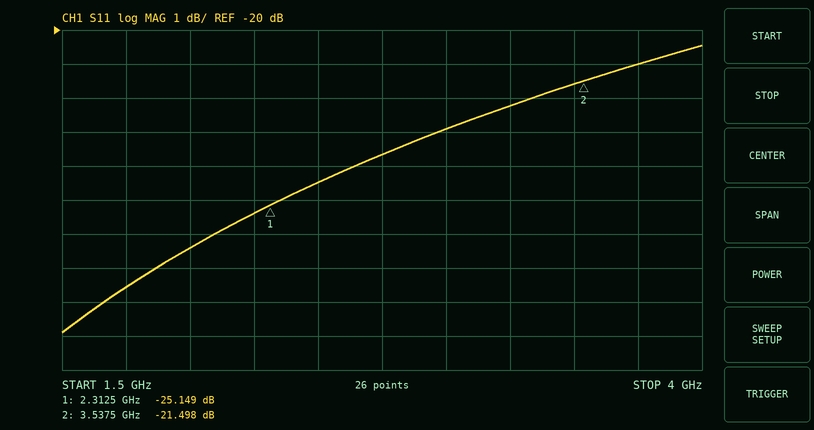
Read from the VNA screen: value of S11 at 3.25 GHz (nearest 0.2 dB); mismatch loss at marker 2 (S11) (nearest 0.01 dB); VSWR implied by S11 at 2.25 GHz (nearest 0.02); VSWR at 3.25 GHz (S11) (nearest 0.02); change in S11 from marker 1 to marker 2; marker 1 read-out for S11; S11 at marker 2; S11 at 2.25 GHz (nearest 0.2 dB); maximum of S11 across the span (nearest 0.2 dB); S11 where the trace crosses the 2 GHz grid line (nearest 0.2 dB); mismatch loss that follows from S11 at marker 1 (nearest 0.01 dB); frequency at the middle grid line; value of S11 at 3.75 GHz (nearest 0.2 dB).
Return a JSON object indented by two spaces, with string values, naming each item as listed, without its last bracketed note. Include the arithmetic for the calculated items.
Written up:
{
  "value of S11 at 3.25 GHz": "-22.2 dB",
  "mismatch loss at marker 2 (S11)": "−10 log10(1 − 10^(-21.498/10)) ≈ 0.03 dB",
  "VSWR implied by S11 at 2.25 GHz": "|Γ| = 10^(-25.4/20) = 0.0537; VSWR = (1 + 0.0537)/(1 − 0.0537) ≈ 1.11, so 1.12 to the nearest 0.02",
  "VSWR at 3.25 GHz (S11)": "|Γ| = 10^(-22.2/20) = 0.0776; VSWR = (1 + 0.0776)/(1 − 0.0776) ≈ 1.17, so 1.16 to the nearest 0.02",
  "change in S11 from marker 1 to marker 2": "-21.498 − (-25.149) = 3.651 dB",
  "marker 1 read-out for S11": "-25.149 dB",
  "S11 at marker 2": "-21.498 dB",
  "S11 at 2.25 GHz": "-25.4 dB",
  "maximum of S11 across the span": "-20.4 dB",
  "S11 where the trace crosses the 2 GHz grid line": "-26.4 dB",
  "mismatch loss that follows from S11 at marker 1": "−10 log10(1 − 10^(-25.149/10)) ≈ 0.01 dB",
  "frequency at the middle grid line": "2.75 GHz",
  "value of S11 at 3.75 GHz": "-21.0 dB"
}
